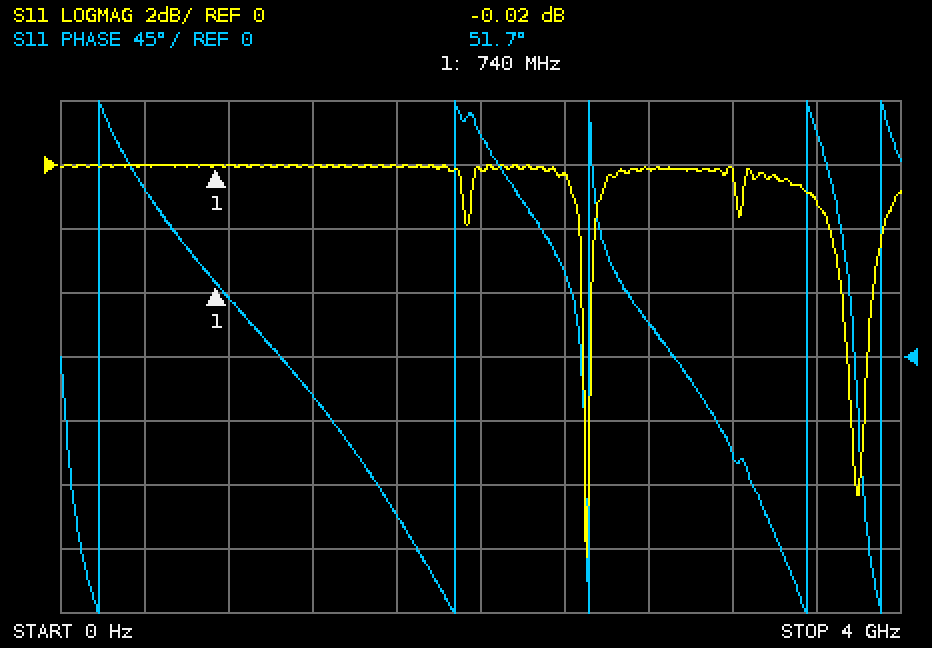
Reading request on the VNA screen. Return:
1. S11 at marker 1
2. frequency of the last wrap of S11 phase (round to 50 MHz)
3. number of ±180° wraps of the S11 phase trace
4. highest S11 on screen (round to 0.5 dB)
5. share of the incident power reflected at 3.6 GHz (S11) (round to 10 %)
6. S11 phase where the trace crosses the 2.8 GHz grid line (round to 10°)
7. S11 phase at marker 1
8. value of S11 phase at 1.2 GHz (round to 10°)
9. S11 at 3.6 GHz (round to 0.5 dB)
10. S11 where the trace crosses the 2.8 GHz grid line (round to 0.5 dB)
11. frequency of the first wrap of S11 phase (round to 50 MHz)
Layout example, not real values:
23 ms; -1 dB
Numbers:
-0.02 dB; 3.90 GHz; 5; 0.0 dB; 80 %; 20°; 51.7°; -30°; -1.0 dB; 0.0 dB; 200 MHz
